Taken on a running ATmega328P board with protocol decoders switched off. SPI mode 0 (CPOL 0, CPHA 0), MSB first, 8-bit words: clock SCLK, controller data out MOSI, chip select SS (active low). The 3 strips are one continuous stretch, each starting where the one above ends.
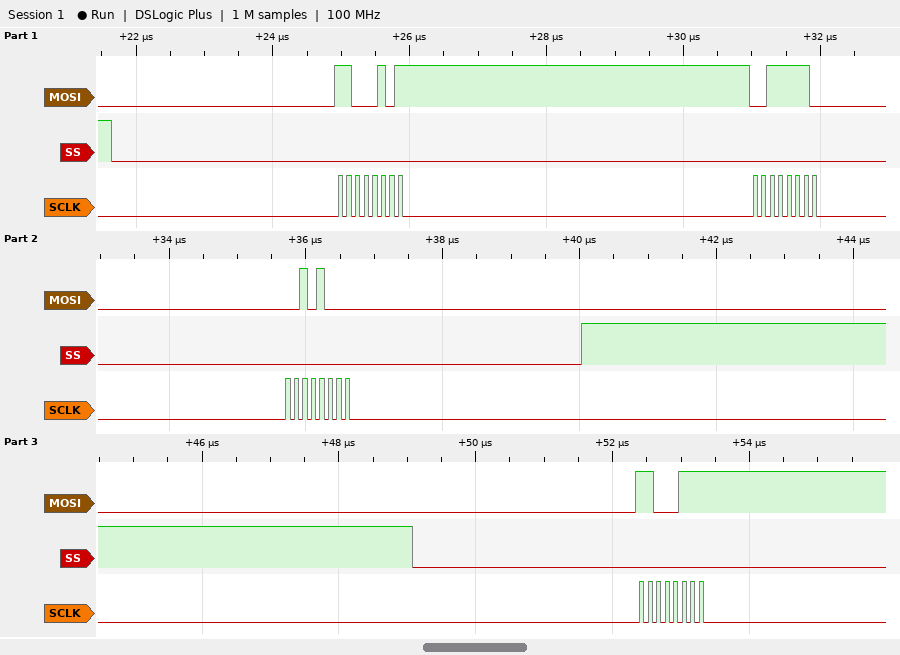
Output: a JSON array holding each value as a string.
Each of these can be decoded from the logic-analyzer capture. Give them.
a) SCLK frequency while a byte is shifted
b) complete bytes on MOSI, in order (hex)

["8 MHz", "C5 3E 28 C7"]
